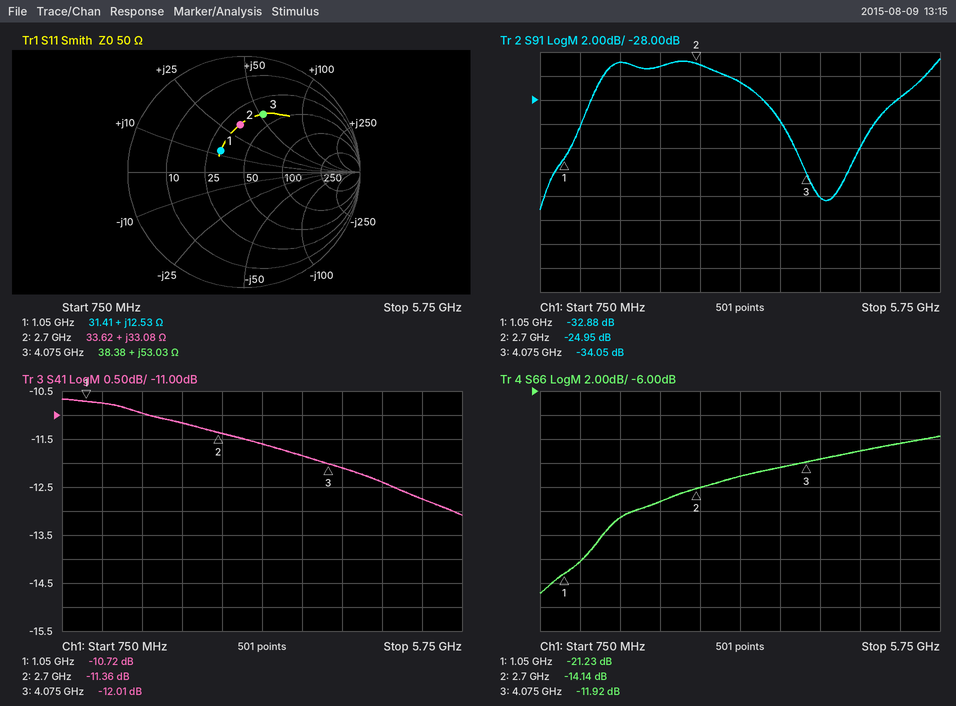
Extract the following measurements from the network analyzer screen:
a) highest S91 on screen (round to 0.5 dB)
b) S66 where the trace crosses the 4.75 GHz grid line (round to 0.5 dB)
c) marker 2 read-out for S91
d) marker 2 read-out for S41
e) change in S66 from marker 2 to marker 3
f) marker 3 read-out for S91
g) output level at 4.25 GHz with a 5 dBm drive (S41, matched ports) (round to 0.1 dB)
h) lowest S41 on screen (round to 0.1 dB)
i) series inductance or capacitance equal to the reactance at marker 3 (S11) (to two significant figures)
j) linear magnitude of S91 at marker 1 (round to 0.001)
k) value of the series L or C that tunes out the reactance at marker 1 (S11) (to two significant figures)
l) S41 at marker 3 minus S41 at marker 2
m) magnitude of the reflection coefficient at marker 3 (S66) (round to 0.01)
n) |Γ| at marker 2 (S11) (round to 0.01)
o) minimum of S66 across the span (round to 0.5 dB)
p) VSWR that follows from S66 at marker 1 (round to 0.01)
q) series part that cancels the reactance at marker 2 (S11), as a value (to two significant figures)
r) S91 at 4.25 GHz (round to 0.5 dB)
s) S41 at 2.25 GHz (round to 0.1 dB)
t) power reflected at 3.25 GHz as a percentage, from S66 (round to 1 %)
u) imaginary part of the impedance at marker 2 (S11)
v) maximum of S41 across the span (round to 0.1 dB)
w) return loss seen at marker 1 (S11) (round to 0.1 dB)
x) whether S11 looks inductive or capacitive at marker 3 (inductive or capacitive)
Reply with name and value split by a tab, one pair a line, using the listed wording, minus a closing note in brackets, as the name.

highest S91 on screen	-24.5 dB
S66 where the trace crosses the 4.75 GHz grid line	-11.0 dB
marker 2 read-out for S91	-24.95 dB
marker 2 read-out for S41	-11.36 dB
change in S66 from marker 2 to marker 3	2.22 dB
marker 3 read-out for S91	-34.05 dB
output level at 4.25 GHz with a 5 dBm drive (S41, matched ports)	-7.1 dBm
lowest S41 on screen	-13.1 dB
series inductance or capacitance equal to the reactance at marker 3 (S11)	2.1 nH
linear magnitude of S91 at marker 1	0.023
value of the series L or C that tunes out the reactance at marker 1 (S11)	12 pF
S41 at marker 3 minus S41 at marker 2	-0.65 dB
magnitude of the reflection coefficient at marker 3 (S66)	0.25
|Γ| at marker 2 (S11)	0.41
minimum of S66 across the span	-23.0 dB
VSWR that follows from S66 at marker 1	1.19
series part that cancels the reactance at marker 2 (S11), as a value	1.8 pF
S91 at 4.25 GHz	-36.0 dB
S41 at 2.25 GHz	-11.2 dB
power reflected at 3.25 GHz as a percentage, from S66	5 %
imaginary part of the impedance at marker 2	+33.08 Ω
maximum of S41 across the span	-10.7 dB
return loss seen at marker 1 (S11)	11.3 dB
whether S11 looks inductive or capacitive at marker 3	inductive
